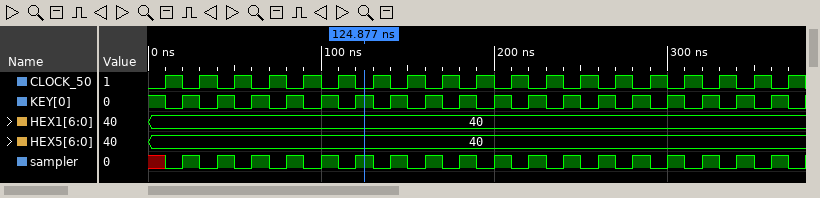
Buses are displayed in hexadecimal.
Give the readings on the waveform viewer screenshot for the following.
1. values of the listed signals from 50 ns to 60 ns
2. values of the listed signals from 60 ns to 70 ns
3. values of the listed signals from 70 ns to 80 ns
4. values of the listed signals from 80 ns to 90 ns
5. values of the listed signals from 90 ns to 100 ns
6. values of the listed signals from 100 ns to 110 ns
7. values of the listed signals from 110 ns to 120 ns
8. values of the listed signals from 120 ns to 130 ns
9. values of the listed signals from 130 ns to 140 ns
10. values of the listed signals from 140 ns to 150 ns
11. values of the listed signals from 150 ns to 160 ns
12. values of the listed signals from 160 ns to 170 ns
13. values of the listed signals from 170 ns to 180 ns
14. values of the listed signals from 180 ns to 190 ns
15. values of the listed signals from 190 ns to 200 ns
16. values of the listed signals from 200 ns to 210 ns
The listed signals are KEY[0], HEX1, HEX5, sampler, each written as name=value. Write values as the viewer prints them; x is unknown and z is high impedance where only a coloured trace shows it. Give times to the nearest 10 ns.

KEY[0]=0, HEX1=40, HEX5=40, sampler=0
KEY[0]=1, HEX1=40, HEX5=40, sampler=1
KEY[0]=0, HEX1=40, HEX5=40, sampler=0
KEY[0]=1, HEX1=40, HEX5=40, sampler=1
KEY[0]=0, HEX1=40, HEX5=40, sampler=0
KEY[0]=1, HEX1=40, HEX5=40, sampler=1
KEY[0]=0, HEX1=40, HEX5=40, sampler=0
KEY[0]=1, HEX1=40, HEX5=40, sampler=1
KEY[0]=0, HEX1=40, HEX5=40, sampler=0
KEY[0]=1, HEX1=40, HEX5=40, sampler=1
KEY[0]=0, HEX1=40, HEX5=40, sampler=0
KEY[0]=1, HEX1=40, HEX5=40, sampler=1
KEY[0]=0, HEX1=40, HEX5=40, sampler=0
KEY[0]=1, HEX1=40, HEX5=40, sampler=1
KEY[0]=0, HEX1=40, HEX5=40, sampler=0
KEY[0]=1, HEX1=40, HEX5=40, sampler=1
